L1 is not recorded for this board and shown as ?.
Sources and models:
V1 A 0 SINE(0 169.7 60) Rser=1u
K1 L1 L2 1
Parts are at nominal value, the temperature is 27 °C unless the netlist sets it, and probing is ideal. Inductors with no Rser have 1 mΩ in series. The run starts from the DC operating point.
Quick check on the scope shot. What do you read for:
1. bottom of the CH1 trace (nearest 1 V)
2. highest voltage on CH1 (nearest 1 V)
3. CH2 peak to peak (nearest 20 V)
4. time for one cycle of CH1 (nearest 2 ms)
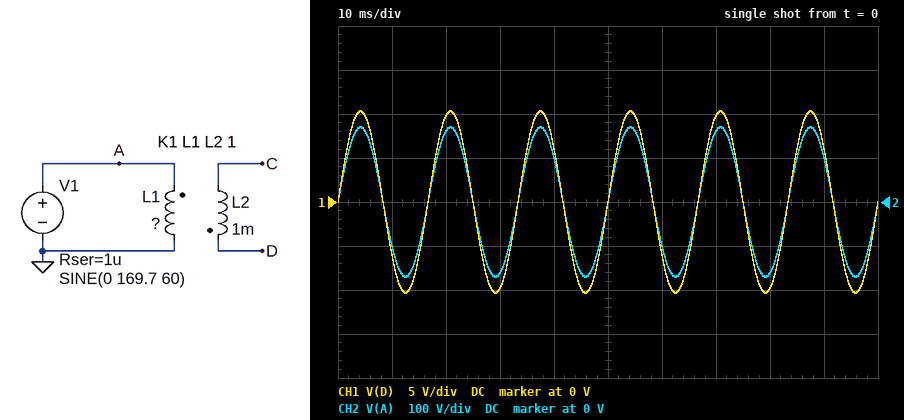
-10 V
10 V
340 V
16 ms
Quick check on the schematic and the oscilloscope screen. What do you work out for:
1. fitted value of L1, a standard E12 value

270 mH
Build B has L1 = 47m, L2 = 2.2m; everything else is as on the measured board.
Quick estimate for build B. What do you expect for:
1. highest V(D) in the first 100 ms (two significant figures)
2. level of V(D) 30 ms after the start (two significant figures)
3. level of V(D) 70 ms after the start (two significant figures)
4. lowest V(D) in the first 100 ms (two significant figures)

37 V
-35 V
35 V
-37 V
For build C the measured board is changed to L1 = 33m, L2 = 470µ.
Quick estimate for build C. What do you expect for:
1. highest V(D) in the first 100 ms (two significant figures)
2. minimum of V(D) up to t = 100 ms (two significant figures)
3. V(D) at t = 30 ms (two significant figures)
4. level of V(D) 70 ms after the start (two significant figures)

20 V
-20 V
-19 V
19 V
